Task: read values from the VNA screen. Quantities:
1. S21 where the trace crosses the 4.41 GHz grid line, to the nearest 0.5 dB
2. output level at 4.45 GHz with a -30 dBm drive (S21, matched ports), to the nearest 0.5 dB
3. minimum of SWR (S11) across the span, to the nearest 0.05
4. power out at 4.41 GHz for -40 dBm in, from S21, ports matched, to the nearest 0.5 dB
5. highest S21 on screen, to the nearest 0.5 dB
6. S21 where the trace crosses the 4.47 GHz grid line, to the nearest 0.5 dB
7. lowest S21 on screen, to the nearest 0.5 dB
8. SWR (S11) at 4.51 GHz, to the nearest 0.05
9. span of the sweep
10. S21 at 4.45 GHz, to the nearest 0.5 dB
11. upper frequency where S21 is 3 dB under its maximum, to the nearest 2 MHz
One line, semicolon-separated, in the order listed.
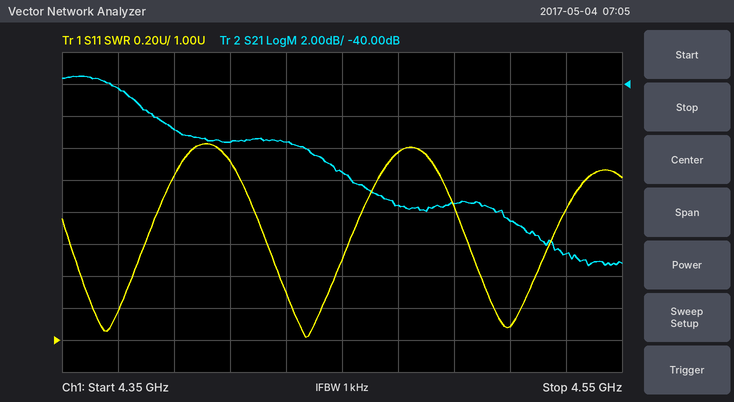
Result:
-43.5 dB; -75.5 dBm; 1.00; -83.5 dBm; -39.5 dB; -47.5 dB; -51.5 dB; 1.10; 200 MHz; -45.5 dB; 4.388 GHz
